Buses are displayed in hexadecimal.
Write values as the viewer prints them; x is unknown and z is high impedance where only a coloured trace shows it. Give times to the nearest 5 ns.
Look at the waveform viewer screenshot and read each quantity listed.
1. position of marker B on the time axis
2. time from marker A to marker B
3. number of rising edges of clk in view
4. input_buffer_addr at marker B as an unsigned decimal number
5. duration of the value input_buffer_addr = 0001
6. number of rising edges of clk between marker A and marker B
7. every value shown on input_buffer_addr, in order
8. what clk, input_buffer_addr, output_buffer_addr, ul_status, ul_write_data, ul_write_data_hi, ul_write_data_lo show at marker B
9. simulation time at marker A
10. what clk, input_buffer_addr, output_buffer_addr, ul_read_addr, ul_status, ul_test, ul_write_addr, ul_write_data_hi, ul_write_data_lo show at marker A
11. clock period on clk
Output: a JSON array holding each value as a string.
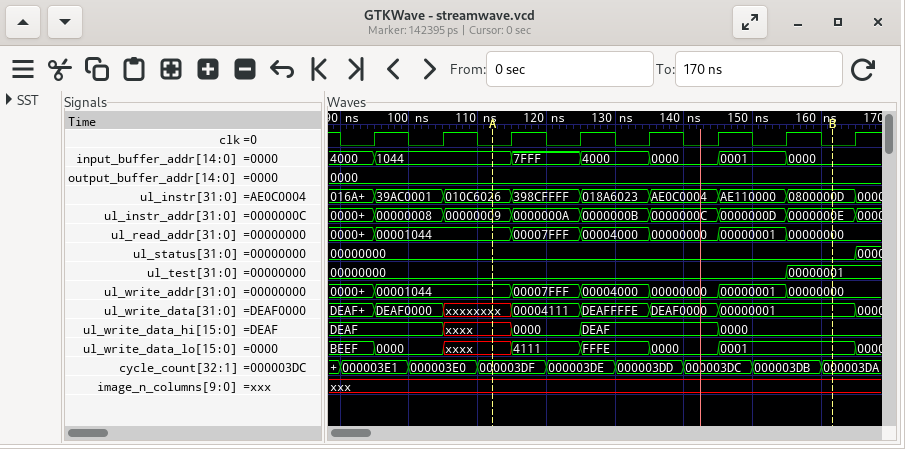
["160 ns", "50 ns", "8", "0", "10 ns", "5", "4000, 1044, 7FFF, 4000, 0000, 0001, 0000", "clk=0, input_buffer_addr=0000, output_buffer_addr=0000, ul_status=00000000, ul_write_data=00000001, ul_write_data_hi=0000, ul_write_data_lo=0001", "110 ns", "clk=0, input_buffer_addr=1044, output_buffer_addr=0000, ul_read_addr=00001044, ul_status=00000000, ul_test=00000000, ul_write_addr=00001044, ul_write_data_hi=xxxx, ul_write_data_lo=xxxx", "10 ns"]
